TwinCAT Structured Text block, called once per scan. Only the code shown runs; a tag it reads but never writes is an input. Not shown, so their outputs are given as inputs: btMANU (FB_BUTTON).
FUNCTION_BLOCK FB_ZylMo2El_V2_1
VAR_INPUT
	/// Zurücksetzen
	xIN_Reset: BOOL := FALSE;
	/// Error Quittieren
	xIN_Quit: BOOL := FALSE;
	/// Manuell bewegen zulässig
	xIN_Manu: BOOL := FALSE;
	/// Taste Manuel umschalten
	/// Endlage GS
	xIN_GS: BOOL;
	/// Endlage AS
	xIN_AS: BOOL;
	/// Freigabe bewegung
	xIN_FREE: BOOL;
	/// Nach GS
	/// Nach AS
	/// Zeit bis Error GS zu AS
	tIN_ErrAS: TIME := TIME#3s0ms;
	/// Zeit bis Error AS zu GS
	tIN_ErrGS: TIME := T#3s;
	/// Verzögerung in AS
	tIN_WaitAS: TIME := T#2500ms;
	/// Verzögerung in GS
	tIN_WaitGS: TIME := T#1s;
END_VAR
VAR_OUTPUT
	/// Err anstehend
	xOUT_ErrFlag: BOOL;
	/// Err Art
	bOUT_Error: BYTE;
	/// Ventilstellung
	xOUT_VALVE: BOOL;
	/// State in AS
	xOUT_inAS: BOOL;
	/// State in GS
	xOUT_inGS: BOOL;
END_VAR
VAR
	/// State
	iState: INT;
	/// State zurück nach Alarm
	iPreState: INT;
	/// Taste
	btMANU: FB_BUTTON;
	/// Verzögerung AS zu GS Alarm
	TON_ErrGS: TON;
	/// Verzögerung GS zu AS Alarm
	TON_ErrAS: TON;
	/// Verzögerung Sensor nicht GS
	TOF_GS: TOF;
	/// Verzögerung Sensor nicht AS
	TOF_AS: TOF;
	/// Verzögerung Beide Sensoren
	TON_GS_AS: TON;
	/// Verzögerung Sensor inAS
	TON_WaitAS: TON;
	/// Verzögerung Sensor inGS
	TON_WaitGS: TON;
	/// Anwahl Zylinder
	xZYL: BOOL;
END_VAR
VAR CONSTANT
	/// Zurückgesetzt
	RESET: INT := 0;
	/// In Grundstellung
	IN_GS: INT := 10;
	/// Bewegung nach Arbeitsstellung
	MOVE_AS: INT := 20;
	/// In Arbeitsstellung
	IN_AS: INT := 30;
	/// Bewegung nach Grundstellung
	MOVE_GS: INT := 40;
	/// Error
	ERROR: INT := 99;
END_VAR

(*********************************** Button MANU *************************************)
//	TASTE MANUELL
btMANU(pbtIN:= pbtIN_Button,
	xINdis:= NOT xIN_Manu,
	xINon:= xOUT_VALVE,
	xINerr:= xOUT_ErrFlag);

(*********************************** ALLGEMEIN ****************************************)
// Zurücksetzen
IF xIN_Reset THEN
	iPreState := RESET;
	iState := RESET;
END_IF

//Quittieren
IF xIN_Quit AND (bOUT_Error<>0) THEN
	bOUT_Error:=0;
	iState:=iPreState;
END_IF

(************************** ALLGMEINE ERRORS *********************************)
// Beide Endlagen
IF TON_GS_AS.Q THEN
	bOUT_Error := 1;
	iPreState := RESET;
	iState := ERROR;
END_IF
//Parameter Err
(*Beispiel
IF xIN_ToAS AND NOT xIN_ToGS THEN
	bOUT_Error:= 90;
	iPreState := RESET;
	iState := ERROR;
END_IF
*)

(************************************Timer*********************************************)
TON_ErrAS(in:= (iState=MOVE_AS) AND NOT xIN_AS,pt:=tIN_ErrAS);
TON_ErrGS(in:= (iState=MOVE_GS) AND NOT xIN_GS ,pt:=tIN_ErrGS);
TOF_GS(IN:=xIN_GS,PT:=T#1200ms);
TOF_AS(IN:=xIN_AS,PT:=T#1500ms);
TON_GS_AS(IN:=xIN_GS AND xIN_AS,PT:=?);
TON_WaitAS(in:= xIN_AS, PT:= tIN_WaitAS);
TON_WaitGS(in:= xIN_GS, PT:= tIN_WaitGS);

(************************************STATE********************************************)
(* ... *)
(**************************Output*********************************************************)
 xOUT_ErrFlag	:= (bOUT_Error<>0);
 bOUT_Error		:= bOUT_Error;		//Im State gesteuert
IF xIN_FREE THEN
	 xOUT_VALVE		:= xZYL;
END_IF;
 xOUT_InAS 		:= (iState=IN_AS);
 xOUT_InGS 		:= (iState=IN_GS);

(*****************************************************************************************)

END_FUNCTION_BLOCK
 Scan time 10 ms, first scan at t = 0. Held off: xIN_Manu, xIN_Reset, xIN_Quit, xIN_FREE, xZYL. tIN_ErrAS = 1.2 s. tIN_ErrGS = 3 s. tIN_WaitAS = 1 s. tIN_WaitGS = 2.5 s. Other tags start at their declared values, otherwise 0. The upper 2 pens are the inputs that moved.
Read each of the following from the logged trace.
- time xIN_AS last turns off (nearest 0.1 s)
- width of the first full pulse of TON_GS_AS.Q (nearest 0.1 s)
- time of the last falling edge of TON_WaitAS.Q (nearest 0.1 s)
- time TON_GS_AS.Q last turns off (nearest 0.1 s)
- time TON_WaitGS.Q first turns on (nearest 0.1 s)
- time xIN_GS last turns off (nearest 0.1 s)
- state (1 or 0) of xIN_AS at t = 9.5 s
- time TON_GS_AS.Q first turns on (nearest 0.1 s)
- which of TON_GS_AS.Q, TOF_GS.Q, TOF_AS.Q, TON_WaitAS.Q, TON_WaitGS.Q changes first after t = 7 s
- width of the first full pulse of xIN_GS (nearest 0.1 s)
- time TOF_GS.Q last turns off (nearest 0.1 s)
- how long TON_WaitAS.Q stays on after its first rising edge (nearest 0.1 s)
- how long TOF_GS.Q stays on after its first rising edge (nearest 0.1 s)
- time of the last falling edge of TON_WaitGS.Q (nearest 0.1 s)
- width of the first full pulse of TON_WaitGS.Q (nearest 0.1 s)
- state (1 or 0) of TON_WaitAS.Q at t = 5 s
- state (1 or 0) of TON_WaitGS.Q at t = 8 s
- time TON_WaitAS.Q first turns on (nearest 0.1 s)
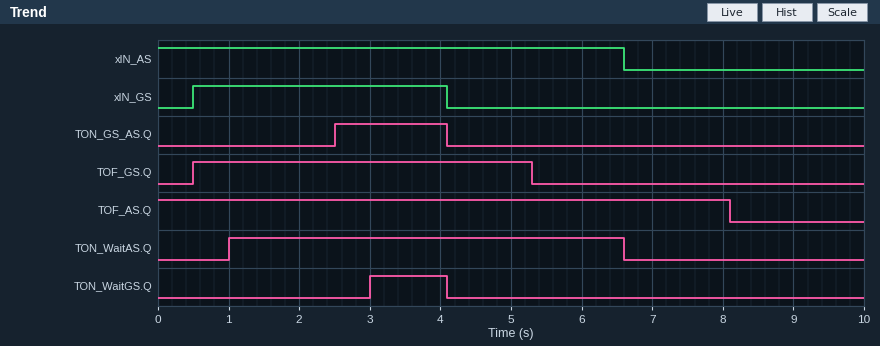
6.6 s
1.6 s
6.6 s
4.1 s
3.0 s
4.1 s
0
2.5 s
TOF_AS.Q
3.6 s
5.3 s
5.6 s
4.8 s
4.1 s
1.1 s
1
0
1.0 s
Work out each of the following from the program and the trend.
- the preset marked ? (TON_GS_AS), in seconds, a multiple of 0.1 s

2.0 s
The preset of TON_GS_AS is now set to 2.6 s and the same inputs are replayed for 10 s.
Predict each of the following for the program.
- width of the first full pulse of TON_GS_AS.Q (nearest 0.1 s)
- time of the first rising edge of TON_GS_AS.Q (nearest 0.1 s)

1.0 s
3.1 s
